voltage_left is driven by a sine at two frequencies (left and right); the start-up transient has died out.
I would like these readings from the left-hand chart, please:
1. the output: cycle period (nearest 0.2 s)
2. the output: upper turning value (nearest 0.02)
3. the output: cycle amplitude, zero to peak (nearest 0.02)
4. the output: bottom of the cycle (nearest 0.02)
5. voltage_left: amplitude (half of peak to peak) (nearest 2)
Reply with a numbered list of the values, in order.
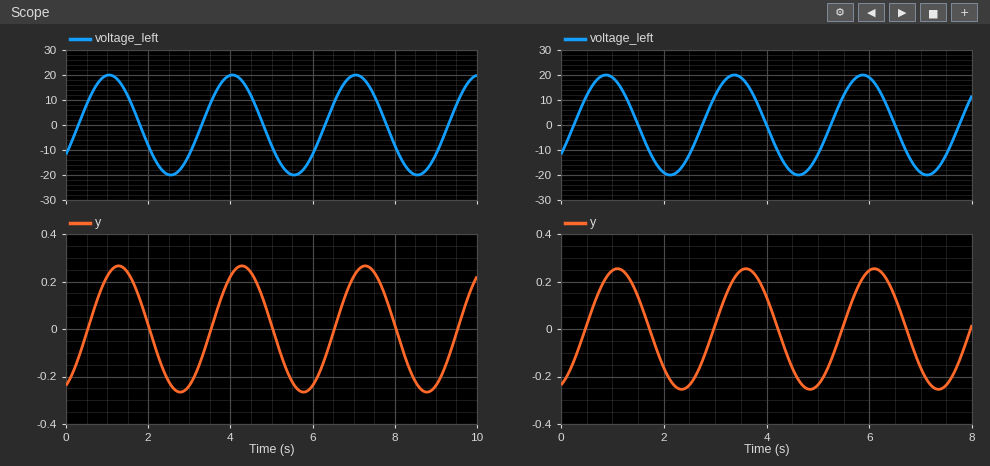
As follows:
1. 3.0 s
2. 0.26
3. 0.26
4. -0.26
5. 20
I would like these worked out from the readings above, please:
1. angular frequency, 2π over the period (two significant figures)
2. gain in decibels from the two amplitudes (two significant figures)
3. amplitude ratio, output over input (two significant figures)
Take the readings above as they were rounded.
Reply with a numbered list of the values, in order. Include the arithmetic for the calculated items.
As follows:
1. 2π / 3 = 2.1 rad/s
2. 20 log10(0.26 / 20) = -38 dB
3. 0.26 / 20 = 0.013
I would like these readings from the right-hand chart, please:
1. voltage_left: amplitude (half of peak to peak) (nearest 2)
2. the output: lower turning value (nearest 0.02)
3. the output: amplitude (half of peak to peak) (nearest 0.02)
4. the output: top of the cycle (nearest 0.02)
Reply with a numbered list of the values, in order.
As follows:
1. 20
2. -0.26
3. 0.26
4. 0.26
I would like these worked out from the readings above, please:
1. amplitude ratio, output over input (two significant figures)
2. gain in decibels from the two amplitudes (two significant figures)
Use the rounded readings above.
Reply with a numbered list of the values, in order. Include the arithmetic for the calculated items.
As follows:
1. 0.26 / 20 = 0.013
2. 20 log10(0.26 / 20) = -38 dB
